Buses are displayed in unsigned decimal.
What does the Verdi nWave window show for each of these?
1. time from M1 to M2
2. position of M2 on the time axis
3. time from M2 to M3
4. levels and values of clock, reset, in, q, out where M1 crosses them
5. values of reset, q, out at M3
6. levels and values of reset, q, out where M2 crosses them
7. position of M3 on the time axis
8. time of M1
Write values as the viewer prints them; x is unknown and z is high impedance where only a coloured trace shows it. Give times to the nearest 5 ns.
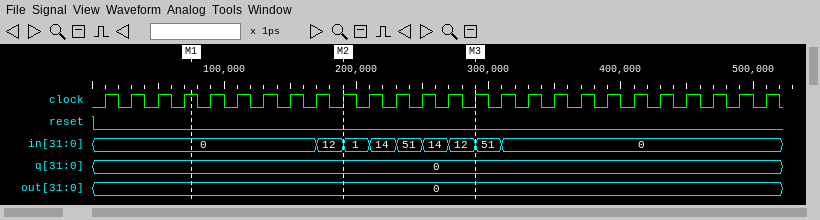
115 ns
190 ns
100 ns
clock=1, reset=0, in=0, q=0, out=0
reset=0, q=0, out=0
reset=0, q=0, out=0
290 ns
75 ns
